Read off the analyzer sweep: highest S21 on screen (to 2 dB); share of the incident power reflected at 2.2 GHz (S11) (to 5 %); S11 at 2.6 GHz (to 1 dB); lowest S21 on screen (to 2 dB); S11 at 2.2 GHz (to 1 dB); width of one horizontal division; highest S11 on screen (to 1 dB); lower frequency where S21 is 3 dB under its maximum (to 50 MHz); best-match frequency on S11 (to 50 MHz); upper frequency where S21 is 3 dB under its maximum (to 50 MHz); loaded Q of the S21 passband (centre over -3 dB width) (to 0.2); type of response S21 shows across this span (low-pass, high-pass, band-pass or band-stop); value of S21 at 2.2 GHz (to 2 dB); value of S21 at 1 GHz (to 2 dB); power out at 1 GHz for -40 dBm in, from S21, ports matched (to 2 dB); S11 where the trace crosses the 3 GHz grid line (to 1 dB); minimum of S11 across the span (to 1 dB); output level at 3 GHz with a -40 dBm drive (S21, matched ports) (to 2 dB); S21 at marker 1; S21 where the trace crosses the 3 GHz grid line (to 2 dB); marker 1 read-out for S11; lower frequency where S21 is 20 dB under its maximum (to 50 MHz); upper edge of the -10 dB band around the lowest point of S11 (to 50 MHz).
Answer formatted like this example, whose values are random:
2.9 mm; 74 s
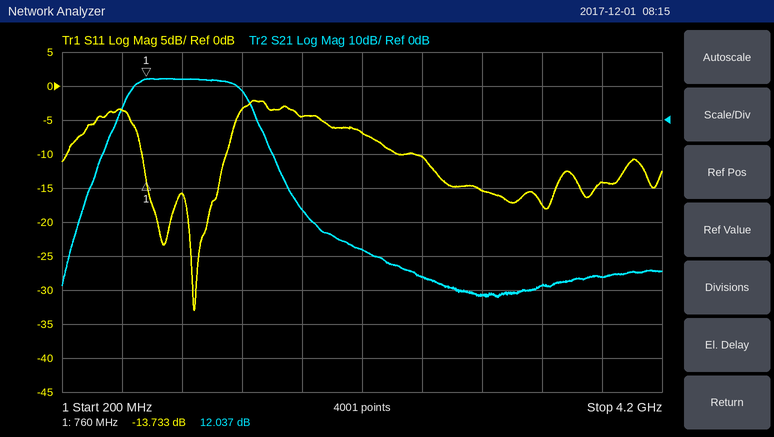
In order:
12 dB; 20 %; -10 dB; -52 dB; -7 dB; 400 MHz; -2 dB; 650 MHz; 1.10 GHz; 1.40 GHz; 1.4; band-pass; -38 dB; 12 dB; -28 dBm; -15 dB; -33 dB; -92 dBm; 12.037 dB; -52 dB; -13.733 dB; 500 MHz; 1.30 GHz
